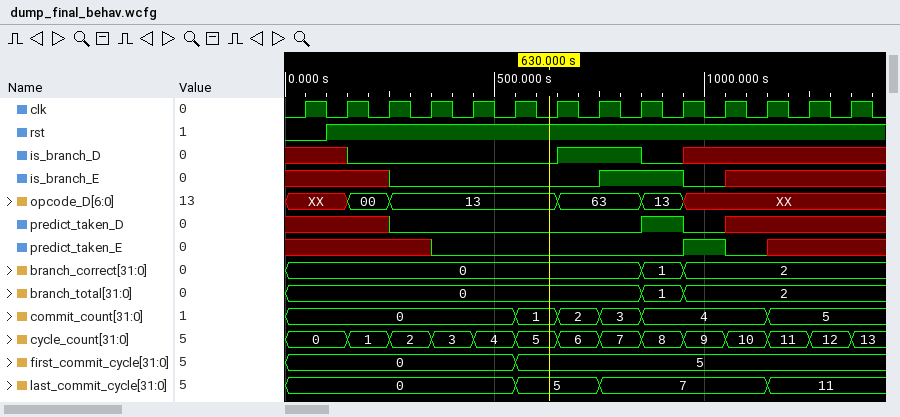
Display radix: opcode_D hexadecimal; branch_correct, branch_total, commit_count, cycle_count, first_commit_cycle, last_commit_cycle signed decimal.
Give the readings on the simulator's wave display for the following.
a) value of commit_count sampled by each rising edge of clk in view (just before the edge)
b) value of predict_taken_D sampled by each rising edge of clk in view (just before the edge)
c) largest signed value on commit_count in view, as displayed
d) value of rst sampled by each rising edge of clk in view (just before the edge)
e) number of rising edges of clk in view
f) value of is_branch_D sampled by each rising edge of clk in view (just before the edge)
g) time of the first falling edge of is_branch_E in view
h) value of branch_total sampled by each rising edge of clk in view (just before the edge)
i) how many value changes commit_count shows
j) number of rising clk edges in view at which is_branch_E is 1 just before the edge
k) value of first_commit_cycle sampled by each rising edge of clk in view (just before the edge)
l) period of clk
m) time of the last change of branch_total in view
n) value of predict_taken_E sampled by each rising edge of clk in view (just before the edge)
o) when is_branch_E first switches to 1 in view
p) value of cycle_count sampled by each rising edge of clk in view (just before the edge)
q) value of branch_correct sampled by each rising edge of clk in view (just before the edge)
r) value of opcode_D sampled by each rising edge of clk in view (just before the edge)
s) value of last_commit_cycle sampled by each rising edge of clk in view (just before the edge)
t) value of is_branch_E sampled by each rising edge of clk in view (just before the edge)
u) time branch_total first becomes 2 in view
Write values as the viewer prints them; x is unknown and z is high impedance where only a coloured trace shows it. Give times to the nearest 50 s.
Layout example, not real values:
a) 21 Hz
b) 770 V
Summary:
a) 0, 0, 0, 0, 0, 0, 1, 2, 3, 4, 4, 4, 5, 5
b) x x x 0 0 0 0 0 0 1 0 x x x
c) 5
d) 0 1 1 1 1 1 1 1 1 1 1 1 1 1
e) 14
f) x x 0 0 0 0 0 1 1 0 x x x x
g) 950 s
h) 0, 0, 0, 0, 0, 0, 0, 0, 0, 1, 2, 2, 2, 2
i) 5
j) 2
k) 0, 0, 0, 0, 0, 0, 5, 5, 5, 5, 5, 5, 5, 5
l) 100 s
m) 950 s
n) x x x x 0 0 0 0 0 0 1 0 x x
o) 750 s
p) 0, 0, 1, 2, 3, 4, 5, 6, 7, 8, 9, 10, 11, 12
q) 0, 0, 0, 0, 0, 0, 0, 0, 0, 1, 2, 2, 2, 2
r) XX, XX, 00, 13, 13, 13, 13, 63, 63, 13, XX, XX, XX, XX
s) 0, 0, 0, 0, 0, 0, 5, 5, 7, 7, 7, 7, 11, 11
t) x x x 0 0 0 0 0 1 1 0 x x x
u) 950 s
